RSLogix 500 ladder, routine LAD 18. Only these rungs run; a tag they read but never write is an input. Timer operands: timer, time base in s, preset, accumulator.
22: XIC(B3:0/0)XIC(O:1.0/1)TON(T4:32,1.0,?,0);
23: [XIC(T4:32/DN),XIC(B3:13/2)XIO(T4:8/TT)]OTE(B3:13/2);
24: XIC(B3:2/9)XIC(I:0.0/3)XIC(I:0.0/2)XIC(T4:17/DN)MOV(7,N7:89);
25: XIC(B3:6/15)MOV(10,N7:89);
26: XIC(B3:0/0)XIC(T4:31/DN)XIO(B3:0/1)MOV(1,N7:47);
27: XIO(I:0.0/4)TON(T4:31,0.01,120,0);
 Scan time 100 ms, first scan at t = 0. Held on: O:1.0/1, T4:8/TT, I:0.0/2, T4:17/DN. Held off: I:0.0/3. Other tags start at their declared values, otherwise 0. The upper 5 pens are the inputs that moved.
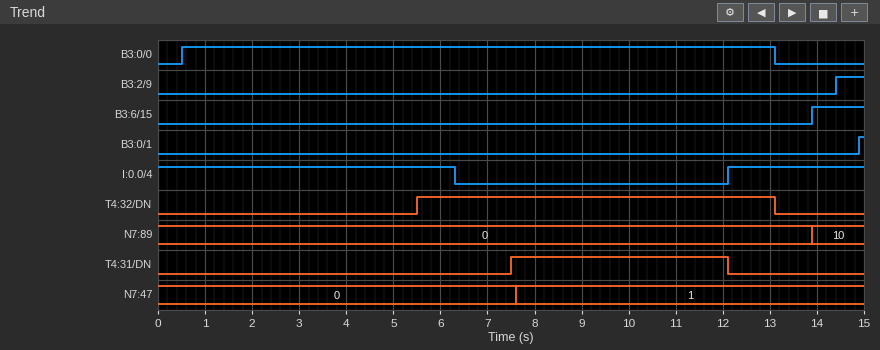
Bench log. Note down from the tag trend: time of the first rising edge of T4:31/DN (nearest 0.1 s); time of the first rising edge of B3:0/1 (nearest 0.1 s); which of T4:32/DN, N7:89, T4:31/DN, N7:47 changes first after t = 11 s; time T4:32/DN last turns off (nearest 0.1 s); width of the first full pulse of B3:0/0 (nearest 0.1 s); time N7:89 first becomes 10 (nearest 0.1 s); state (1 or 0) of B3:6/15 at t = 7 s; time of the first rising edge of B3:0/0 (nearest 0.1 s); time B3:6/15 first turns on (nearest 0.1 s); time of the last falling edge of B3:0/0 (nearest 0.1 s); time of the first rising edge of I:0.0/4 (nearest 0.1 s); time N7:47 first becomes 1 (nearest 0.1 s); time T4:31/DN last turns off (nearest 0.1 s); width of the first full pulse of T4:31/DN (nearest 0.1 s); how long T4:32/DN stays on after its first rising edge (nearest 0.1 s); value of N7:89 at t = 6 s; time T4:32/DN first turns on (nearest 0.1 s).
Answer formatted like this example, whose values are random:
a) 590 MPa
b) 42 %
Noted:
a) 7.5 s
b) 14.9 s
c) T4:31/DN
d) 13.1 s
e) 12.6 s
f) 13.9 s
g) 0
h) 0.5 s
i) 13.9 s
j) 13.1 s
k) 12.1 s
l) 7.6 s
m) 12.1 s
n) 4.6 s
o) 7.6 s
p) 0
q) 5.5 s
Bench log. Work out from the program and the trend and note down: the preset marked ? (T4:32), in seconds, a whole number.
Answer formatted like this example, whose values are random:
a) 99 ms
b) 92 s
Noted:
a) 5 s
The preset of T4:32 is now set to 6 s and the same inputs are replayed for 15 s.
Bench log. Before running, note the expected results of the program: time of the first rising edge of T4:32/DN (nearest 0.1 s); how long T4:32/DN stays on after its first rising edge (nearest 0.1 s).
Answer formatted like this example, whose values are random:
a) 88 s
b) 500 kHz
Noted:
a) 6.5 s
b) 6.6 s
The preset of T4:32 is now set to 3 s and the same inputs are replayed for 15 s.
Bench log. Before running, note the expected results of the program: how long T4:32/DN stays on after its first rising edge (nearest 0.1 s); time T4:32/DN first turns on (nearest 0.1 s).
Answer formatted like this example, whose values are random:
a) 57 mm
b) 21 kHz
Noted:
a) 9.6 s
b) 3.5 s
